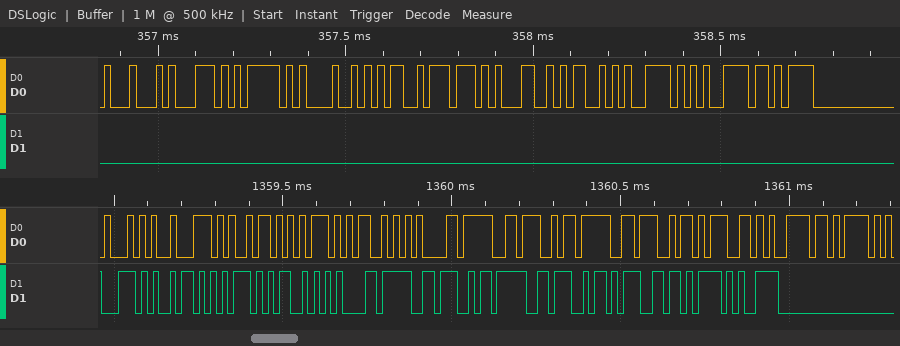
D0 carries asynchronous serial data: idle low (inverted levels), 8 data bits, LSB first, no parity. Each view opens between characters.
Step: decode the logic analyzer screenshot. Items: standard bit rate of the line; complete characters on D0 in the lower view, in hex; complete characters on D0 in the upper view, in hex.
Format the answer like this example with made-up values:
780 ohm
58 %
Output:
57600 baud
57, 47, 4B, 45, 59, 3D, 30, 2C, 30, 2C, 31, 0D, 0A
77, 47, 41, 6F, 65, 44, 67, 59, 43, 0D, 0A
